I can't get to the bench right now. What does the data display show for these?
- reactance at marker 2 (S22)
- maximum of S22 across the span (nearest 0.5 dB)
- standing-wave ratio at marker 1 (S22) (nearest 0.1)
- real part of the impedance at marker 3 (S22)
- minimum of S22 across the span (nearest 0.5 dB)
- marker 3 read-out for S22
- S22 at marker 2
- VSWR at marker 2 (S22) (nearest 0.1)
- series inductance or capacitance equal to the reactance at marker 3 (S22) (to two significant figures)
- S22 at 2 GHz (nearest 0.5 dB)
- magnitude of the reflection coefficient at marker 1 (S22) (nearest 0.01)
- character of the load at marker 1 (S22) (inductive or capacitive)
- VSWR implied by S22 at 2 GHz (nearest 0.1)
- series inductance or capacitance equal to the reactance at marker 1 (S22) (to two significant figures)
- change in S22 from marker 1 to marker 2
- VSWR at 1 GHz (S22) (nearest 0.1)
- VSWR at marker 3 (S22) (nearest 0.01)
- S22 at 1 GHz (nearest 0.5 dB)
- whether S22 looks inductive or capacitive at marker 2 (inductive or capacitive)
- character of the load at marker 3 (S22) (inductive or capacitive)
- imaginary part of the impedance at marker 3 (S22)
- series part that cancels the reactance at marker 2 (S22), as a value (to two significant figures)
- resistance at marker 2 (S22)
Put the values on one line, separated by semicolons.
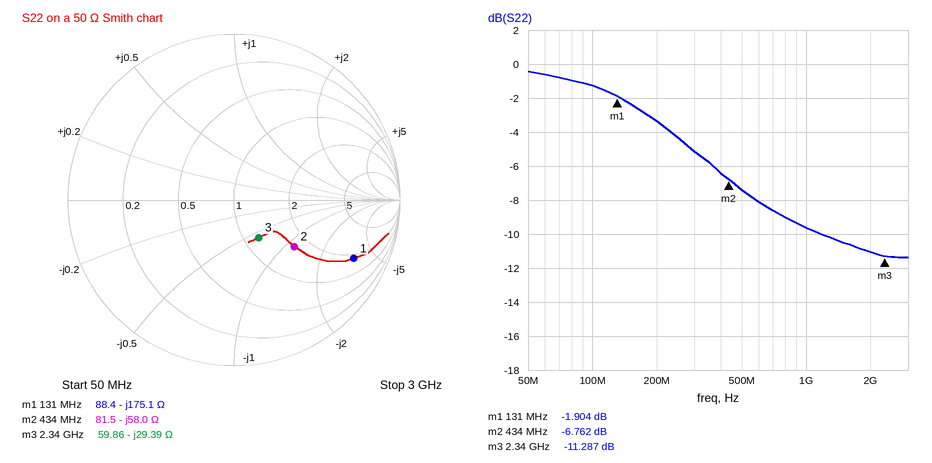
-58.0 Ω; -0.5 dB; 9.2; 59.86 Ω; -11.5 dB; -11.287 dB; -6.762 dB; 2.7; 2.3 pF; -11.0 dB; 0.80; capacitive; 1.8; 6.9 pF; -4.858 dB; 2.0; 1.75; -9.5 dB; capacitive; capacitive; -29.39 Ω; 21 nH; 81.5 Ω
